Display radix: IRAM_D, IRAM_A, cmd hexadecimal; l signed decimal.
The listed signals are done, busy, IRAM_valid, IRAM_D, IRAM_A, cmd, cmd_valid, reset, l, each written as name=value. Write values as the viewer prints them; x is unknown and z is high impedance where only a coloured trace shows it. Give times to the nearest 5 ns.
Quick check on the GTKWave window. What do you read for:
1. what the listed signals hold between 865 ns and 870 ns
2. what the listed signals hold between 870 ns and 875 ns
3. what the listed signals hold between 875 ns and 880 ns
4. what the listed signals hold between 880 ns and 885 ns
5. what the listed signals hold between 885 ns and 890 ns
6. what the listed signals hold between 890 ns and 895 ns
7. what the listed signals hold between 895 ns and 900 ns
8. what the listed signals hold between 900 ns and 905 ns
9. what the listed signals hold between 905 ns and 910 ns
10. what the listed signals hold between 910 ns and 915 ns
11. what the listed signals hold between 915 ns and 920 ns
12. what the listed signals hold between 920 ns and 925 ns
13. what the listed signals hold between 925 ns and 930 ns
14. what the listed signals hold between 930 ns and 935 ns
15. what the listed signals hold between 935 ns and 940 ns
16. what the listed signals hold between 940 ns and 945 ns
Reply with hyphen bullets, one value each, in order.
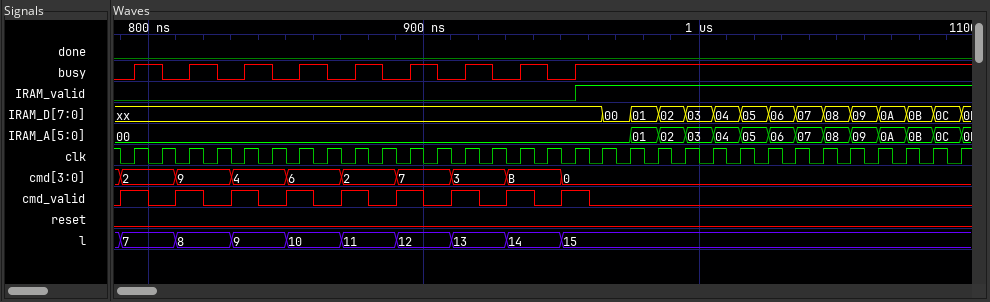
- done=0, busy=0, IRAM_valid=0, IRAM_D=xx, IRAM_A=00, cmd=6, cmd_valid=0, reset=0, l=10
- done=0, busy=0, IRAM_valid=0, IRAM_D=xx, IRAM_A=00, cmd=2, cmd_valid=1, reset=0, l=11
- done=0, busy=1, IRAM_valid=0, IRAM_D=xx, IRAM_A=00, cmd=2, cmd_valid=1, reset=0, l=11
- done=0, busy=1, IRAM_valid=0, IRAM_D=xx, IRAM_A=00, cmd=2, cmd_valid=0, reset=0, l=11
- done=0, busy=0, IRAM_valid=0, IRAM_D=xx, IRAM_A=00, cmd=2, cmd_valid=0, reset=0, l=11
- done=0, busy=0, IRAM_valid=0, IRAM_D=xx, IRAM_A=00, cmd=7, cmd_valid=1, reset=0, l=12
- done=0, busy=1, IRAM_valid=0, IRAM_D=xx, IRAM_A=00, cmd=7, cmd_valid=1, reset=0, l=12
- done=0, busy=1, IRAM_valid=0, IRAM_D=xx, IRAM_A=00, cmd=7, cmd_valid=0, reset=0, l=12
- done=0, busy=0, IRAM_valid=0, IRAM_D=xx, IRAM_A=00, cmd=7, cmd_valid=0, reset=0, l=12
- done=0, busy=0, IRAM_valid=0, IRAM_D=xx, IRAM_A=00, cmd=3, cmd_valid=1, reset=0, l=13
- done=0, busy=1, IRAM_valid=0, IRAM_D=xx, IRAM_A=00, cmd=3, cmd_valid=1, reset=0, l=13
- done=0, busy=1, IRAM_valid=0, IRAM_D=xx, IRAM_A=00, cmd=3, cmd_valid=0, reset=0, l=13
- done=0, busy=0, IRAM_valid=0, IRAM_D=xx, IRAM_A=00, cmd=3, cmd_valid=0, reset=0, l=13
- done=0, busy=0, IRAM_valid=0, IRAM_D=xx, IRAM_A=00, cmd=B, cmd_valid=1, reset=0, l=14
- done=0, busy=1, IRAM_valid=0, IRAM_D=xx, IRAM_A=00, cmd=B, cmd_valid=1, reset=0, l=14
- done=0, busy=1, IRAM_valid=0, IRAM_D=xx, IRAM_A=00, cmd=B, cmd_valid=0, reset=0, l=14
